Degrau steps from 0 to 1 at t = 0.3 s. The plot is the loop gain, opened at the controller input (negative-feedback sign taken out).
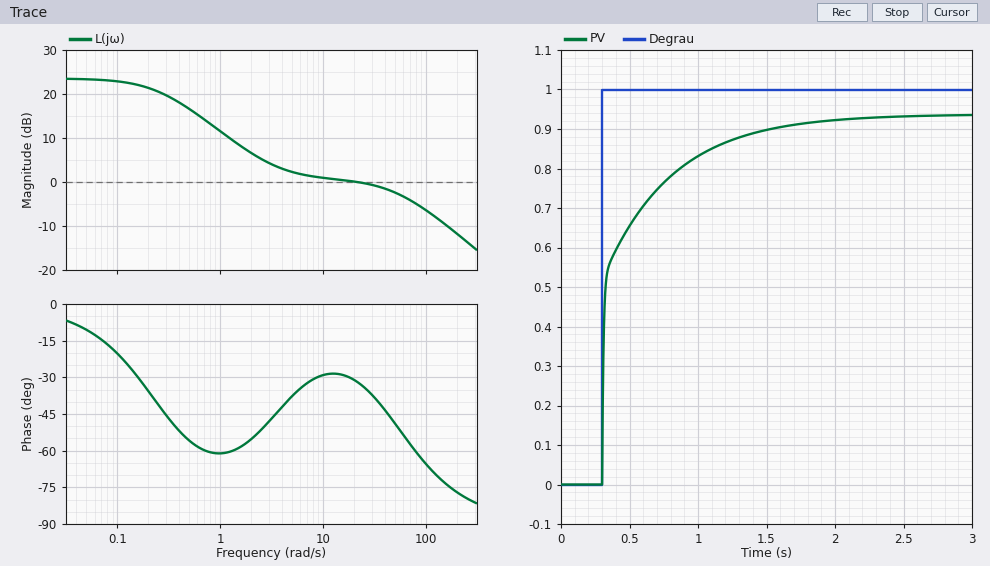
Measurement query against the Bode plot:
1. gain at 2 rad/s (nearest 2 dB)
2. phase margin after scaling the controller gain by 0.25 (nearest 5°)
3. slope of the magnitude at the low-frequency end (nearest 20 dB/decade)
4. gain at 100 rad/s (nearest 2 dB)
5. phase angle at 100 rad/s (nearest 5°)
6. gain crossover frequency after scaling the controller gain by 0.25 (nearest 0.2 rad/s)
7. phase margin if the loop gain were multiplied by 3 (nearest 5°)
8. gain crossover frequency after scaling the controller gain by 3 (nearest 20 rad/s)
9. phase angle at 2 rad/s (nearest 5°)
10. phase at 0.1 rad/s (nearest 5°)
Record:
6 dB
120°
0 dB/decade
-6 dB
-65°
1.0 rad/s
105°
160 rad/s
-55°
-20°
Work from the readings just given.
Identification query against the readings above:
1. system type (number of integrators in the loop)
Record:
0
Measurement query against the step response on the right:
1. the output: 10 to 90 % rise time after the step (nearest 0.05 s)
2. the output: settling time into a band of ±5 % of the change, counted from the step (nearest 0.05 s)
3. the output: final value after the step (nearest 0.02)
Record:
0.75 s
1.10 s
0.94
